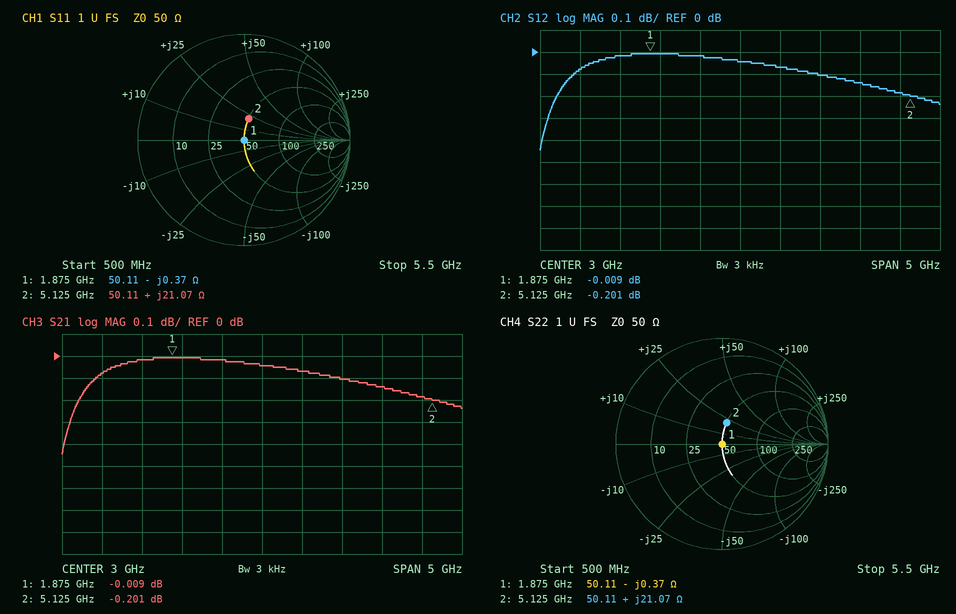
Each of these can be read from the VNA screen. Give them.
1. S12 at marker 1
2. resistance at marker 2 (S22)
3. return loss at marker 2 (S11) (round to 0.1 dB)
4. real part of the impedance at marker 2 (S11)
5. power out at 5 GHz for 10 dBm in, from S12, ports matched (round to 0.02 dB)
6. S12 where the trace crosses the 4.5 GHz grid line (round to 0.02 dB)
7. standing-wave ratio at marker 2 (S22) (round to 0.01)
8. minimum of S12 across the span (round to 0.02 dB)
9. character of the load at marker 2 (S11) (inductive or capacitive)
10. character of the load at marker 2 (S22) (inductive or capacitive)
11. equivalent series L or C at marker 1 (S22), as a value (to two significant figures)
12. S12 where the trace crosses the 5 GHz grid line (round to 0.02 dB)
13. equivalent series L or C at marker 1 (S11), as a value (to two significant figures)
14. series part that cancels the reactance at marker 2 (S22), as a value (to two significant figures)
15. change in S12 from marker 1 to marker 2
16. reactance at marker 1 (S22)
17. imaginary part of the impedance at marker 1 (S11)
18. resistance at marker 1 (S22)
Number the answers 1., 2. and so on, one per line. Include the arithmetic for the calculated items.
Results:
1. -0.009 dB
2. 50.11 Ω
3. 13.7 dB
4. 50.11 Ω
5. 10 dBm + (-0.18 dB) = 9.82 dBm
6. -0.14 dB
7. 1.52
8. -0.44 dB
9. inductive
10. inductive
11. C = 1/(2π × 1.875 GHz × 0.37 Ω) ≈ 229 pF, so 230 pF to two significant figures
12. -0.18 dB
13. C = 1/(2π × 1.875 GHz × 0.37 Ω) ≈ 229 pF, so 230 pF to two significant figures
14. C = 1/(2π × 5.125 GHz × 21.07 Ω) ≈ 1.5 pF
15. -0.201 − (-0.009) = -0.192 dB
16. -0.37 Ω
17. -0.37 Ω
18. 50.11 Ω
